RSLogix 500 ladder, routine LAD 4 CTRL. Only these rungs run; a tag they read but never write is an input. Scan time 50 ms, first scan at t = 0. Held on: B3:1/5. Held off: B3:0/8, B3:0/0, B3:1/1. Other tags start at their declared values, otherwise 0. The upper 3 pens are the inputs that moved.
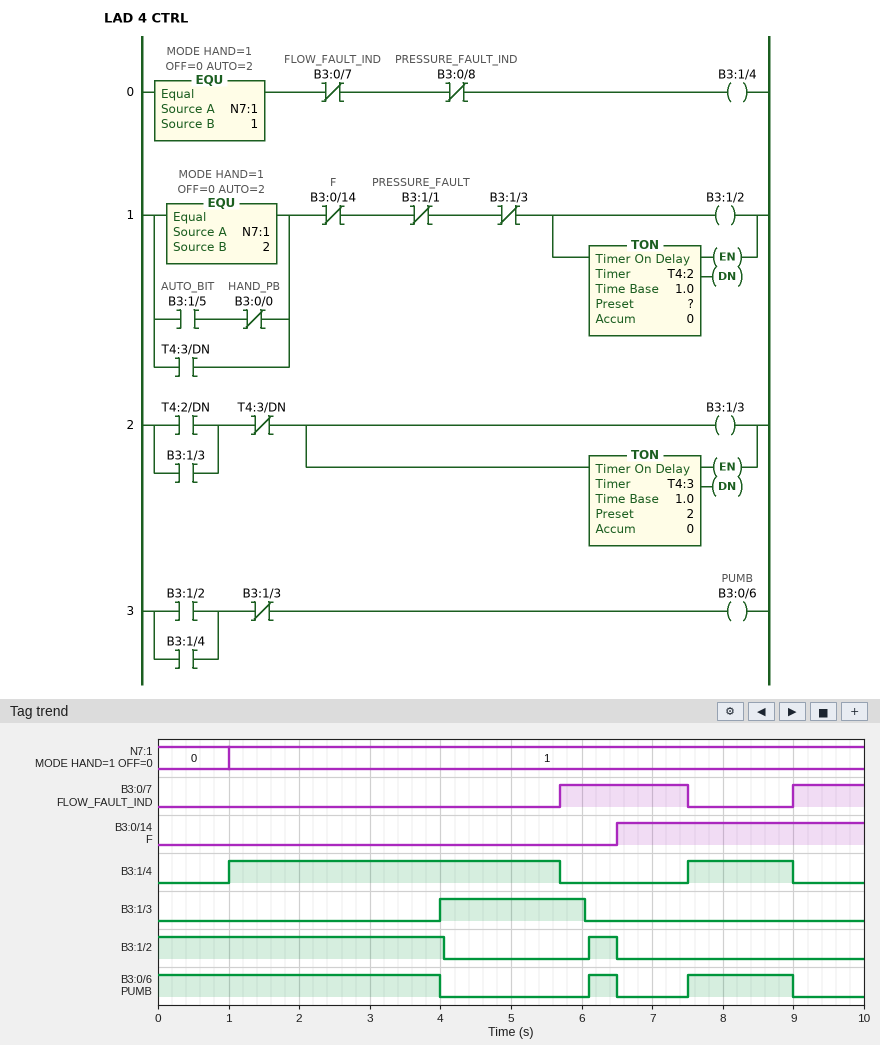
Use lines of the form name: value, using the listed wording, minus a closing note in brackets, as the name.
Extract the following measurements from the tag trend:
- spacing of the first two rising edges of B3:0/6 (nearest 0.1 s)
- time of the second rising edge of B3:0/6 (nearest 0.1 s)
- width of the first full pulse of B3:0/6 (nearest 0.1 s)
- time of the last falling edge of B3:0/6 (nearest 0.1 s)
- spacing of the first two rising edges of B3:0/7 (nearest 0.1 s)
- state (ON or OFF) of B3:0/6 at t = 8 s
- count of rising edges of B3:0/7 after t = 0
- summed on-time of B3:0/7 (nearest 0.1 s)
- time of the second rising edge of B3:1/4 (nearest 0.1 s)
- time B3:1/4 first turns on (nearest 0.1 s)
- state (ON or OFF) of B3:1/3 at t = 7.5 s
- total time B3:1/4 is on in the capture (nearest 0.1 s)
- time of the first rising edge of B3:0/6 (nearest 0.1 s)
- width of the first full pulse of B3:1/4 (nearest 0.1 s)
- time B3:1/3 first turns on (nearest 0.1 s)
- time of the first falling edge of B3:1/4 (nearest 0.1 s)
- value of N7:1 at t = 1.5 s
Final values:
spacing of the first two rising edges of B3:0/6: 1.4 s
time of the second rising edge of B3:0/6: 7.5 s
width of the first full pulse of B3:0/6: 0.4 s
time of the last falling edge of B3:0/6: 9.0 s
spacing of the first two rising edges of B3:0/7: 3.3 s
state (ON or OFF) of B3:0/6 at t = 8 s: ON
count of rising edges of B3:0/7 after t = 0: 2
summed on-time of B3:0/7: 2.8 s
time of the second rising edge of B3:1/4: 7.5 s
time B3:1/4 first turns on: 1.0 s
state (ON or OFF) of B3:1/3 at t = 7.5 s: OFF
total time B3:1/4 is on in the capture: 6.2 s
time of the first rising edge of B3:0/6: 6.1 s
width of the first full pulse of B3:1/4: 4.7 s
time B3:1/3 first turns on: 4.0 s
time of the first falling edge of B3:1/4: 5.7 s
value of N7:1 at t = 1.5 s: 1
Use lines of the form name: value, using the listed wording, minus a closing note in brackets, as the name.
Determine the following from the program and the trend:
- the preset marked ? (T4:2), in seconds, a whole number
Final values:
the preset marked ? (T4:2), in seconds, a whole number: 4 s
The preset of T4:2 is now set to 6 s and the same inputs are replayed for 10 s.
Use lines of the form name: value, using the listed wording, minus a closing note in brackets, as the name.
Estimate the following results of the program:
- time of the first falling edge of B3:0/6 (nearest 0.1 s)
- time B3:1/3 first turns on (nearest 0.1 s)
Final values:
time of the first falling edge of B3:0/6: 6.0 s
time B3:1/3 first turns on: 6.0 s
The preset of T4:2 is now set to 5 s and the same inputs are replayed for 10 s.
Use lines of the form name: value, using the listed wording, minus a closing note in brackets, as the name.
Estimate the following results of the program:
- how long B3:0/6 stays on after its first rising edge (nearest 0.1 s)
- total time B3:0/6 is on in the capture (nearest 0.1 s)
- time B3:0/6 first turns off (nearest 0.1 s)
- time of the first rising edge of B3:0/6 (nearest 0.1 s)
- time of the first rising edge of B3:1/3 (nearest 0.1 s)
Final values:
how long B3:0/6 stays on after its first rising edge: 1.5 s
total time B3:0/6 is on in the capture: 6.5 s
time B3:0/6 first turns off: 5.0 s
time of the first rising edge of B3:0/6: 7.5 s
time of the first rising edge of B3:1/3: 5.0 s
